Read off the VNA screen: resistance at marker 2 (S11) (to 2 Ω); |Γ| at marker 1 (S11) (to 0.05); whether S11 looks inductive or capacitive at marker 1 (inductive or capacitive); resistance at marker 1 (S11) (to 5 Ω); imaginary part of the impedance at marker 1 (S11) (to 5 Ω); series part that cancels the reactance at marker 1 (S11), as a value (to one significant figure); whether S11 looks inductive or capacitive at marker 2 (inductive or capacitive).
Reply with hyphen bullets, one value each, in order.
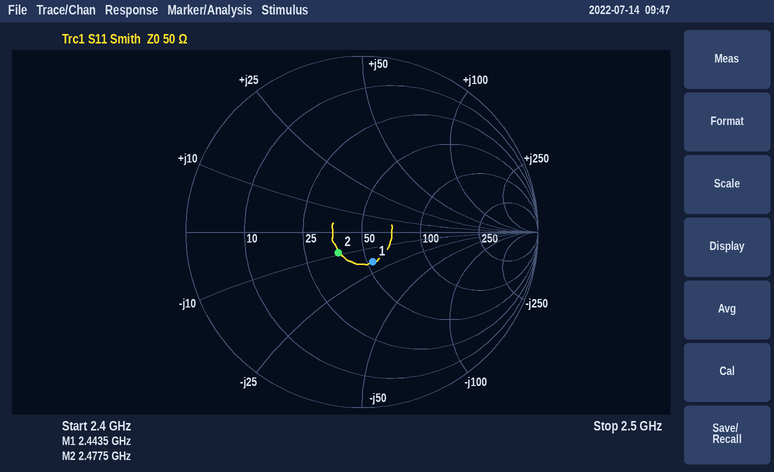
- 38 Ω
- 0.20
- capacitive
- 55 Ω
- -20 Ω
- 1 nH
- capacitive
